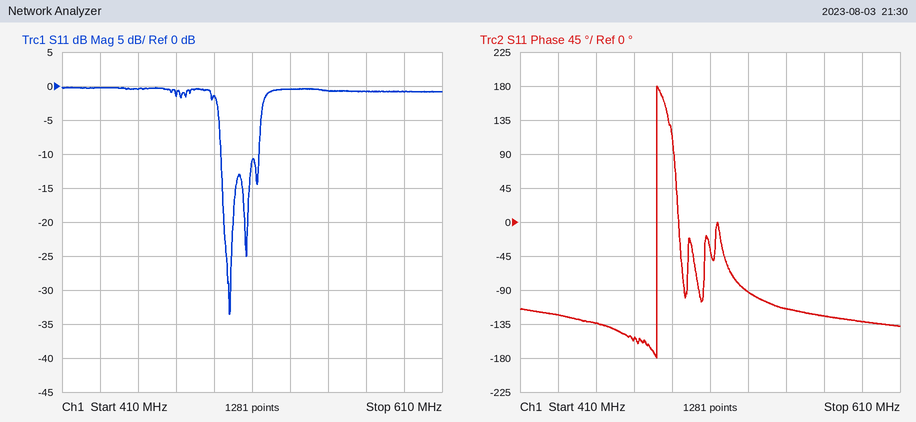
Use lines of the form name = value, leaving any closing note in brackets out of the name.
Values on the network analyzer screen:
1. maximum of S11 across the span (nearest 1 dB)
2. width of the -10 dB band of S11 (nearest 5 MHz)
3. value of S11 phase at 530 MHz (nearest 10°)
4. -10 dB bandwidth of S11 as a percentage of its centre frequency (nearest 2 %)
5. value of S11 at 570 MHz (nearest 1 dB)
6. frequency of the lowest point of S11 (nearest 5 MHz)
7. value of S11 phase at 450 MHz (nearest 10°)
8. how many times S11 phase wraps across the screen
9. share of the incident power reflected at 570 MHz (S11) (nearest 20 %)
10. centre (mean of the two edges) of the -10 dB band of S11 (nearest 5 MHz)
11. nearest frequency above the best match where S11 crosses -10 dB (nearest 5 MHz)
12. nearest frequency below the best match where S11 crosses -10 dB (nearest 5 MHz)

maximum of S11 across the span = 0 dB
width of the -10 dB band of S11 = 20 MHz
value of S11 phase at 530 MHz = -90°
-10 dB bandwidth of S11 as a percentage of its centre frequency = 4 %
value of S11 at 570 MHz = -1 dB
frequency of the lowest point of S11 = 500 MHz
value of S11 phase at 450 MHz = -130°
how many times S11 phase wraps across the screen = 1
share of the incident power reflected at 570 MHz (S11) = 80 %
centre (mean of the two edges) of the -10 dB band of S11 = 505 MHz
nearest frequency above the best match where S11 crosses -10 dB = 515 MHz
nearest frequency below the best match where S11 crosses -10 dB = 495 MHz
